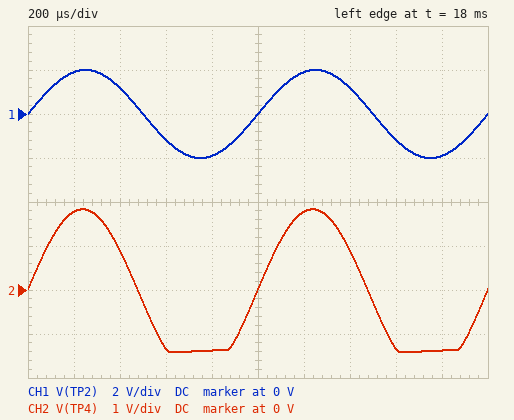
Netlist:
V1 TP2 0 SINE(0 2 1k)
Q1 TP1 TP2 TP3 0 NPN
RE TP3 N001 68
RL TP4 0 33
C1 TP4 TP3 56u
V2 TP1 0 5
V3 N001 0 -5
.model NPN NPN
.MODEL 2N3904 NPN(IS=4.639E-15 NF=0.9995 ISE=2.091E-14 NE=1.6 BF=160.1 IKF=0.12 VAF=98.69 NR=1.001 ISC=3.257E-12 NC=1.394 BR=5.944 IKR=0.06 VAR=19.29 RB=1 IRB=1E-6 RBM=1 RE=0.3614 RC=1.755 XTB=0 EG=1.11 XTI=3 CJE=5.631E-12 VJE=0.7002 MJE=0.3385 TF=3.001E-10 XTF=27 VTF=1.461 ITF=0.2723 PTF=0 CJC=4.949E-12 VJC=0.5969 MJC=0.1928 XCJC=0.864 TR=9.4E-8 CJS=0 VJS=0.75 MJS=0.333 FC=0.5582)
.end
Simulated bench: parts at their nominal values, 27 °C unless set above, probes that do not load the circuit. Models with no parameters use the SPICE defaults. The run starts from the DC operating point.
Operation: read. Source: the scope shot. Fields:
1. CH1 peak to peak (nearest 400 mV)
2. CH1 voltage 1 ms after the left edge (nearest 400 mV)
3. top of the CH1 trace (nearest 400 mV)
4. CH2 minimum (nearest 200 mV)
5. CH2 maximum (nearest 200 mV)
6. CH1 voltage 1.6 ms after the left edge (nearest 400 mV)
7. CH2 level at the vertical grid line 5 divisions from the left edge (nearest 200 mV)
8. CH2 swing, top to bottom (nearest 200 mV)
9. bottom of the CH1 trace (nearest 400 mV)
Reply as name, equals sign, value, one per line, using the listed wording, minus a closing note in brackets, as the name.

CH1 peak to peak = 4.0 V
CH1 voltage 1 ms after the left edge = 0 V
top of the CH1 trace = 2.0 V
CH2 minimum = -1.4 V
CH2 maximum = 1.8 V
CH1 voltage 1.6 ms after the left edge = -1.2 V
CH2 level at the vertical grid line 5 divisions from the left edge = 0 V
CH2 swing, top to bottom = 3.2 V
bottom of the CH1 trace = -2.0 V
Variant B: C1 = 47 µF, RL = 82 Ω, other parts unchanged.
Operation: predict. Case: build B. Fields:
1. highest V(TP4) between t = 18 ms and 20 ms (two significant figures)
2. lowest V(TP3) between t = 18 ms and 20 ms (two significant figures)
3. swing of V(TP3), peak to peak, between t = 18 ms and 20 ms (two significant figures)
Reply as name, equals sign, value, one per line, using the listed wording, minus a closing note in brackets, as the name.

highest V(TP4) between t = 18 ms and 20 ms = 2.0 V
lowest V(TP3) between t = 18 ms and 20 ms = -2.8 V
swing of V(TP3), peak to peak, between t = 18 ms and 20 ms = 3.9 V
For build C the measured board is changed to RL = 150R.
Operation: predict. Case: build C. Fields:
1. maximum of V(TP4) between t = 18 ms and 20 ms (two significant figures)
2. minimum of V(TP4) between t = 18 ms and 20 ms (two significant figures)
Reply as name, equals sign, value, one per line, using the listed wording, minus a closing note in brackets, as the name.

maximum of V(TP4) between t = 18 ms and 20 ms = 2.0 V
minimum of V(TP4) between t = 18 ms and 20 ms = -2.0 V
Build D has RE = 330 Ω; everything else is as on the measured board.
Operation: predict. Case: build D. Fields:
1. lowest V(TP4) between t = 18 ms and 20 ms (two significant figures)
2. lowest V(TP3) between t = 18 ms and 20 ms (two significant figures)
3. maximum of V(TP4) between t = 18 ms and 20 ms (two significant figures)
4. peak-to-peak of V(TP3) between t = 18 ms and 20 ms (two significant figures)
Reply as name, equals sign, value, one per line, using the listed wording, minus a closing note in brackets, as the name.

lowest V(TP4) between t = 18 ms and 20 ms = -460 mV
lowest V(TP3) between t = 18 ms and 20 ms = -530 mV
maximum of V(TP4) between t = 18 ms and 20 ms = 1.1 V
peak-to-peak of V(TP3) between t = 18 ms and 20 ms = 1.7 V
